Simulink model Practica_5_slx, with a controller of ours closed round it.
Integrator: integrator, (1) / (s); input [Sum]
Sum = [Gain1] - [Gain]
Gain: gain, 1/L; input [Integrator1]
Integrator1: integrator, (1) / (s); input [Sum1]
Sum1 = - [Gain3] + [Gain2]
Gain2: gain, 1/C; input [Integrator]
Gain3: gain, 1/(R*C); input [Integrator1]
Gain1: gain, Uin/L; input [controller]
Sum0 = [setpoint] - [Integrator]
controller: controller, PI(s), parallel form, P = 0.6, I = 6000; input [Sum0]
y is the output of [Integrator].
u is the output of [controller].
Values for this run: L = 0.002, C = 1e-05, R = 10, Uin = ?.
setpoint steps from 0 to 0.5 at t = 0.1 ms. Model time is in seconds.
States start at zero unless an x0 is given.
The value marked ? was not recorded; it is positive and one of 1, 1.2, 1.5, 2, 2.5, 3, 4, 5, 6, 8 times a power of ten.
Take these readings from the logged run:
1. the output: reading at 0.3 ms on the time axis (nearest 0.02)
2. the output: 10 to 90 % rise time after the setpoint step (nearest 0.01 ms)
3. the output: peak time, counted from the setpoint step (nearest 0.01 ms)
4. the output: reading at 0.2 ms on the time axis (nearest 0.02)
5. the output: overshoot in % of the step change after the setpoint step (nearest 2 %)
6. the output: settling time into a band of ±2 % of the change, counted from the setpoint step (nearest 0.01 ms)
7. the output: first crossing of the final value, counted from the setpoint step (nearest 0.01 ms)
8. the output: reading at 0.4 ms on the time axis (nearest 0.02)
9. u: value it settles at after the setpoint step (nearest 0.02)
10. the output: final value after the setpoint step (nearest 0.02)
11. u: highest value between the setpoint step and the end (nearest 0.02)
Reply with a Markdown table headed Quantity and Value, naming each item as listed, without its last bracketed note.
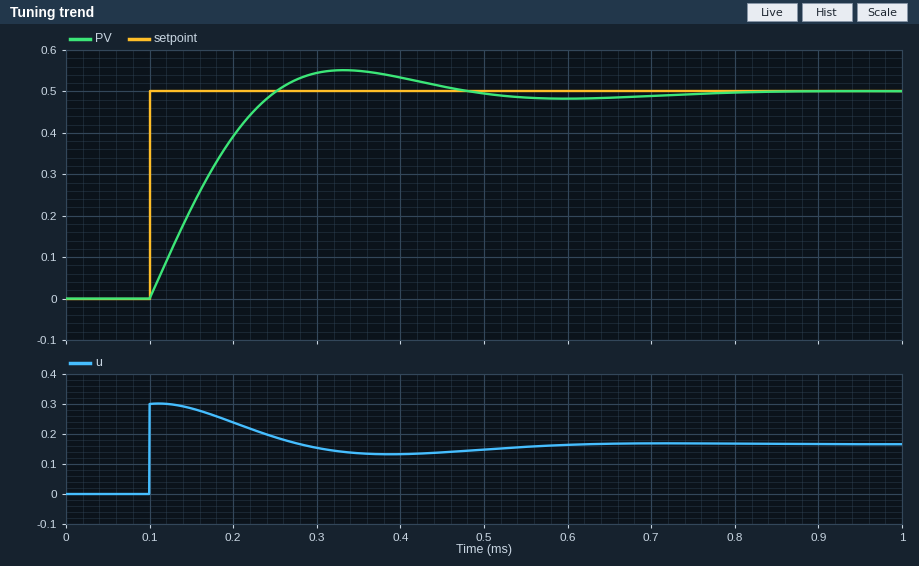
| Quantity | Value |
|---|---|
| the output: reading at 0.3 ms on the time axis | 0.54 |
| the output: 10 to 90 % rise time after the setpoint step | 0.11 ms |
| the output: peak time, counted from the setpoint step | 0.23 ms |
| the output: reading at 0.2 ms on the time axis | 0.40 |
| the output: overshoot in % of the step change after the setpoint step | 10 % |
| the output: settling time into a band of ±2 % of the change, counted from the setpoint step | 0.61 ms |
| the output: first crossing of the final value, counted from the setpoint step | 0.15 ms |
| the output: reading at 0.4 ms on the time axis | 0.54 |
| u: value it settles at after the setpoint step | 0.16 |
| the output: final value after the setpoint step | 0.50 |
| u: highest value between the setpoint step and the end | 0.30 |
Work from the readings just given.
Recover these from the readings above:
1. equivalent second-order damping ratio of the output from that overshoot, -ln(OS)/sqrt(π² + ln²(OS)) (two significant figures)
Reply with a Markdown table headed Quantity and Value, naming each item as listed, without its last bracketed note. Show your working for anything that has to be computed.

| Quantity | Value |
|---|---|
| equivalent second-order damping ratio of the output from that overshoot, -ln(OS)/sqrt(π² + ln²(OS)) | ln(0.1) = -2.303; 2.303 / sqrt(9.870 + 5.302) = 0.59 |
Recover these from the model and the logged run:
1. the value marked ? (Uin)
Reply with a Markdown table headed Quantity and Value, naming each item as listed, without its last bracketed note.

| Quantity | Value |
|---|---|
| the value marked ? | 30 |
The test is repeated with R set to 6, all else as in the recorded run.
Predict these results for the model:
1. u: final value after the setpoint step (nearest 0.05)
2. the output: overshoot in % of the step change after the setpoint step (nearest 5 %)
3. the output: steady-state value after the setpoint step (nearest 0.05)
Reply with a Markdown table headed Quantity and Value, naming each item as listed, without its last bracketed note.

| Quantity | Value |
|---|---|
| u: final value after the setpoint step | 0.10 |
| the output: overshoot in % of the step change after the setpoint step | 15 % |
| the output: steady-state value after the setpoint step | 0.50 |
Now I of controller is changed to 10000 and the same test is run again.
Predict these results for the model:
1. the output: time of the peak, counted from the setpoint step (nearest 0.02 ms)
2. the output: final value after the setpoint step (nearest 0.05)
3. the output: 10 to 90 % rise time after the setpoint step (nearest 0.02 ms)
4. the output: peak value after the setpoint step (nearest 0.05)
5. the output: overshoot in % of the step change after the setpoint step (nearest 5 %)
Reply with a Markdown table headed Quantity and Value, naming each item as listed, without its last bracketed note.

| Quantity | Value |
|---|---|
| the output: time of the peak, counted from the setpoint step | 0.20 ms |
| the output: final value after the setpoint step | 0.50 |
| the output: 10 to 90 % rise time after the setpoint step | 0.08 ms |
| the output: peak value after the setpoint step | 0.60 |
| the output: overshoot in % of the step change after the setpoint step | 20 % |
